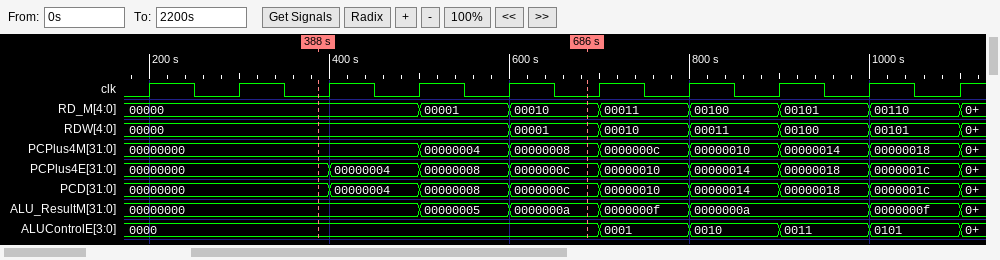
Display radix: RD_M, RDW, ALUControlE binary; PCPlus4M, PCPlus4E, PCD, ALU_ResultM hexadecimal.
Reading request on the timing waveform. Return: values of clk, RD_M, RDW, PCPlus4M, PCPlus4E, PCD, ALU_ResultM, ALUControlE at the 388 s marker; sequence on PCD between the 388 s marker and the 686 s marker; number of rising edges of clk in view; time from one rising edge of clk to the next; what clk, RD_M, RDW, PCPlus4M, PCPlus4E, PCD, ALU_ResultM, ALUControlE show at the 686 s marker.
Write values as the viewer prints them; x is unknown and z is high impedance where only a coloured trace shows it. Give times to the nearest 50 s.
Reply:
clk=0, RD_M=00000, RDW=00000, PCPlus4M=00000000, PCPlus4E=00000000, PCD=00000000, ALU_ResultM=00000000, ALUControlE=0000
00000000, 00000004, 00000008, 0000000c
10
100 s
clk=0, RD_M=00010, RDW=00001, PCPlus4M=00000008, PCPlus4E=0000000c, PCD=0000000c, ALU_ResultM=0000000a, ALUControlE=0000
